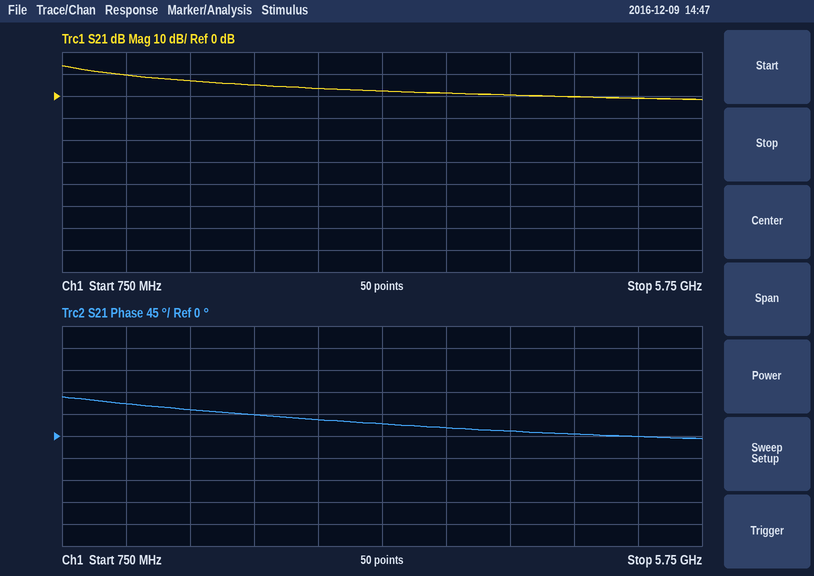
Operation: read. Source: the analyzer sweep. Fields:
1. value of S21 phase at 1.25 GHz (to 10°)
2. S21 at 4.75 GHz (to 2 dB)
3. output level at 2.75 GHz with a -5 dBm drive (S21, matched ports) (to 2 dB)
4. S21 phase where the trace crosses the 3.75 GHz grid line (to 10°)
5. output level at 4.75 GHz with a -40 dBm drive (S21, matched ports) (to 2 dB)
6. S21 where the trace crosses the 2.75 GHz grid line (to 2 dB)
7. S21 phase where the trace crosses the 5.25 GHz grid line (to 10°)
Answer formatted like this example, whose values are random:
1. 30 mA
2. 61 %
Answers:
1. 70°
2. 0 dB
3. -2 dBm
4. 20°
5. -40 dBm
6. 4 dB
7. 0°
